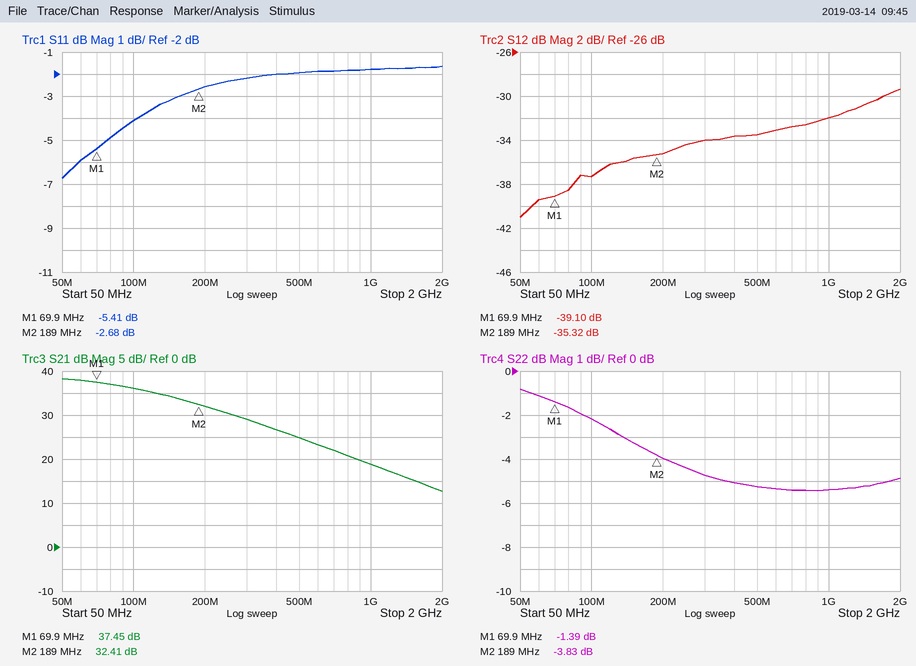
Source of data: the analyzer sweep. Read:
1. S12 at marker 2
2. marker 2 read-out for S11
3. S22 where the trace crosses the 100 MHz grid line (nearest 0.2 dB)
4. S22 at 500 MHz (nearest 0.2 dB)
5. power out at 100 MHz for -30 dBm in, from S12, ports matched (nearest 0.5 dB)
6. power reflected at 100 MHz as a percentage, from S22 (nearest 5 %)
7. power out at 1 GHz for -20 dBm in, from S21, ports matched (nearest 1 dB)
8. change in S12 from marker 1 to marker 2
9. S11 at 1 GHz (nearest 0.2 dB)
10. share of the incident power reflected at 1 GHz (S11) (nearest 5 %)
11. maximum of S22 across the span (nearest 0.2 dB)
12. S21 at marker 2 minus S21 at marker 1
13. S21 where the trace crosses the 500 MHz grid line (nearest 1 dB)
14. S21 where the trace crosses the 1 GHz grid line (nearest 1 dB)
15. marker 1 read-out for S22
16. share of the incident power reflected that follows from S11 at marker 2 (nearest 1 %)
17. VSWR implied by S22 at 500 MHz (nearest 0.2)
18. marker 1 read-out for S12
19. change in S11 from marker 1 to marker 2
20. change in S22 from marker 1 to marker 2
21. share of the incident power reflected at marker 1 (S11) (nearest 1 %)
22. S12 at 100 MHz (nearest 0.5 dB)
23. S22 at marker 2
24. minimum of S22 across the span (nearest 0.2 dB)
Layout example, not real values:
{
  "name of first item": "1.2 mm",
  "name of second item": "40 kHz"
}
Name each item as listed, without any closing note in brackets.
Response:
{
  "S12 at marker 2": "-35.32 dB",
  "marker 2 read-out for S11": "-2.68 dB",
  "S22 where the trace crosses the 100 MHz grid line": "-2.2 dB",
  "S22 at 500 MHz": "-5.2 dB",
  "power out at 100 MHz for -30 dBm in, from S12, ports matched": "-67.5 dBm",
  "power reflected at 100 MHz as a percentage, from S22": "60 %",
  "power out at 1 GHz for -20 dBm in, from S21, ports matched": "-1 dBm",
  "change in S12 from marker 1 to marker 2": "3.78 dB",
  "S11 at 1 GHz": "-1.8 dB",
  "share of the incident power reflected at 1 GHz (S11)": "65 %",
  "maximum of S22 across the span": "-0.8 dB",
  "S21 at marker 2 minus S21 at marker 1": "-5.04 dB",
  "S21 where the trace crosses the 500 MHz grid line": "25 dB",
  "S21 where the trace crosses the 1 GHz grid line": "19 dB",
  "marker 1 read-out for S22": "-1.39 dB",
  "share of the incident power reflected that follows from S11 at marker 2": "54 %",
  "VSWR implied by S22 at 500 MHz": "3.4",
  "marker 1 read-out for S12": "-39.10 dB",
  "change in S11 from marker 1 to marker 2": "2.73 dB",
  "change in S22 from marker 1 to marker 2": "-2.44 dB",
  "share of the incident power reflected at marker 1 (S11)": "29 %",
  "S12 at 100 MHz": "-37.5 dB",
  "S22 at marker 2": "-3.83 dB",
  "minimum of S22 across the span": "-5.4 dB"
}
